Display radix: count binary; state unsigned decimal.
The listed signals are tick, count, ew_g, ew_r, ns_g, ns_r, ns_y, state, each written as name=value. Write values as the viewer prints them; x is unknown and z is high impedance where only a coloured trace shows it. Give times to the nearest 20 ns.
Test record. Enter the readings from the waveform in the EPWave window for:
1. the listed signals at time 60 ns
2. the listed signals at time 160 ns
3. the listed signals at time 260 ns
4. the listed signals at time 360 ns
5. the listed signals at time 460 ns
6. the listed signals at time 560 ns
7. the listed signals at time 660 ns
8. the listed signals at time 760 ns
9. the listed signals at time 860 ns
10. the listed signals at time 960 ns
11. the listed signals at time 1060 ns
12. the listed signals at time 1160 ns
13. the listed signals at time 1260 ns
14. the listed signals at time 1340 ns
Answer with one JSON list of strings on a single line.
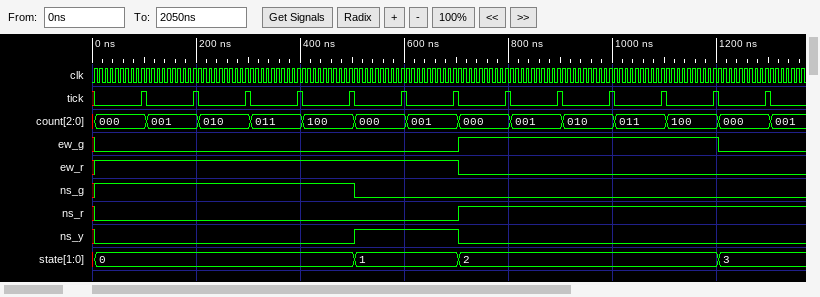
["tick=0, count=000, ew_g=0, ew_r=1, ns_g=1, ns_r=0, ns_y=0, state=0", "tick=0, count=001, ew_g=0, ew_r=1, ns_g=1, ns_r=0, ns_y=0, state=0", "tick=0, count=010, ew_g=0, ew_r=1, ns_g=1, ns_r=0, ns_y=0, state=0", "tick=0, count=011, ew_g=0, ew_r=1, ns_g=1, ns_r=0, ns_y=0, state=0", "tick=0, count=100, ew_g=0, ew_r=1, ns_g=1, ns_r=0, ns_y=0, state=0", "tick=0, count=000, ew_g=0, ew_r=1, ns_g=0, ns_r=0, ns_y=1, state=1", "tick=0, count=001, ew_g=0, ew_r=1, ns_g=0, ns_r=0, ns_y=1, state=1", "tick=0, count=000, ew_g=1, ew_r=0, ns_g=0, ns_r=1, ns_y=0, state=2", "tick=0, count=001, ew_g=1, ew_r=0, ns_g=0, ns_r=1, ns_y=0, state=2", "tick=0, count=010, ew_g=1, ew_r=0, ns_g=0, ns_r=1, ns_y=0, state=2", "tick=0, count=011, ew_g=1, ew_r=0, ns_g=0, ns_r=1, ns_y=0, state=2", "tick=0, count=100, ew_g=1, ew_r=0, ns_g=0, ns_r=1, ns_y=0, state=2", "tick=0, count=000, ew_g=0, ew_r=0, ns_g=0, ns_r=1, ns_y=0, state=3", "tick=0, count=001, ew_g=0, ew_r=0, ns_g=0, ns_r=1, ns_y=0, state=3"]
